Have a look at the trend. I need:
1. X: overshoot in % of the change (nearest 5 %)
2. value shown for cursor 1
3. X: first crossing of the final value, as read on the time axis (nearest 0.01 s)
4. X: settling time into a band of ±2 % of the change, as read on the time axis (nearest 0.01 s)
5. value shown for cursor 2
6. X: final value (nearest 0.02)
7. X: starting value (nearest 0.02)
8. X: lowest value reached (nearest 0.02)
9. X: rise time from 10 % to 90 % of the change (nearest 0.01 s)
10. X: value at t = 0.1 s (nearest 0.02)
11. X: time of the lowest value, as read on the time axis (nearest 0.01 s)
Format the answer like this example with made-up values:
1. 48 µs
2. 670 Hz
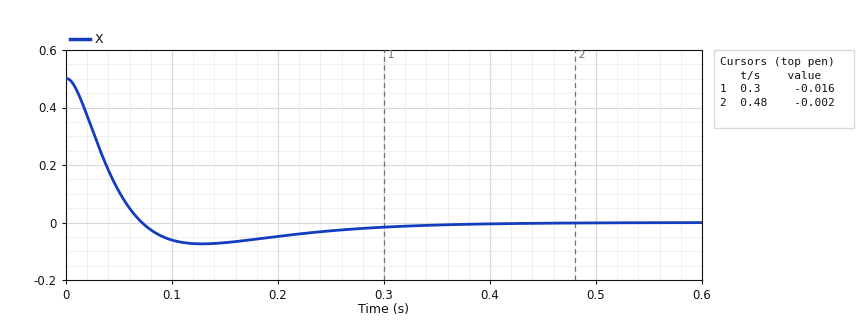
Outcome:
1. 15 %
2. -0.016
3. 0.07 s
4. 0.34 s
5. -0.002
6. 0.00
7. 0.50
8. -0.08
9. 0.05 s
10. -0.06
11. 0.13 s
